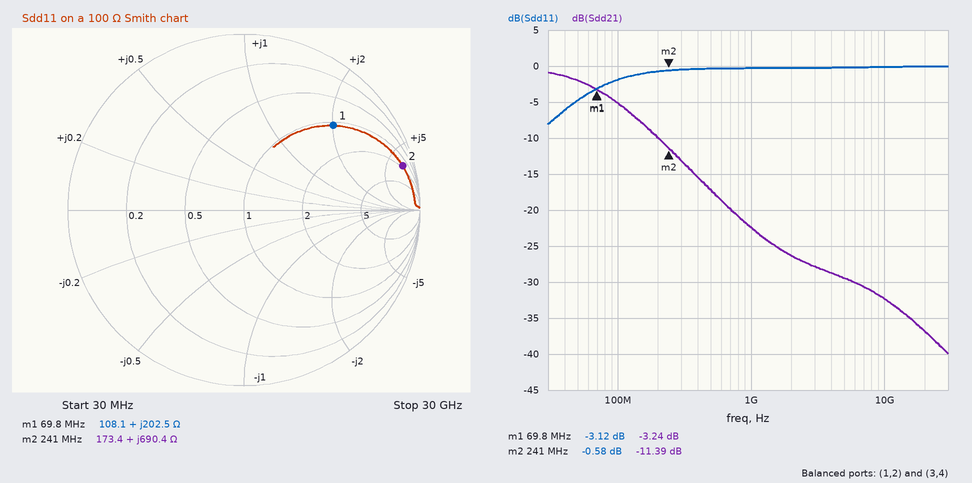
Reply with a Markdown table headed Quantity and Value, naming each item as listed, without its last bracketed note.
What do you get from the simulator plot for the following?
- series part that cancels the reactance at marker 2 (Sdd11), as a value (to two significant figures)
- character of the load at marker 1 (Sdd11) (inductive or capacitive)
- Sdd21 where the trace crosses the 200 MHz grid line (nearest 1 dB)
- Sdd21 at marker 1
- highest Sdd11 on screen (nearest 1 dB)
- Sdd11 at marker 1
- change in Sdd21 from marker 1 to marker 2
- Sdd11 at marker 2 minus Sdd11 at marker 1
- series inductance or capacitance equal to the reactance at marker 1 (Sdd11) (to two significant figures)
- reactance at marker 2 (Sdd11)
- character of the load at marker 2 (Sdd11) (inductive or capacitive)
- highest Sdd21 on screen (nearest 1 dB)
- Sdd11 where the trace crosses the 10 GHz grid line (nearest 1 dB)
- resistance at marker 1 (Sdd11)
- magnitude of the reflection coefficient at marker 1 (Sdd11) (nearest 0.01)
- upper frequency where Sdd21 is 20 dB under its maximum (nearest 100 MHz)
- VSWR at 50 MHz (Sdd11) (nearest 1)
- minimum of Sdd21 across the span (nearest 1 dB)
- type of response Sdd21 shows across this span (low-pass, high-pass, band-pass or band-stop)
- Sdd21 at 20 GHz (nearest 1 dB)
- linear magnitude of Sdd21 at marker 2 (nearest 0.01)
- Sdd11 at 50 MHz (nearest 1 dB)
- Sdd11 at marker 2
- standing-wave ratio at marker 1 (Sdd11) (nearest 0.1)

| Quantity | Value |
|---|---|
| series part that cancels the reactance at marker 2 (Sdd11), as a value | 960 fF |
| character of the load at marker 1 (Sdd11) | inductive |
| Sdd21 where the trace crosses the 200 MHz grid line | -10 dB |
| Sdd21 at marker 1 | -3.24 dB |
| highest Sdd11 on screen | 0 dB |
| Sdd11 at marker 1 | -3.12 dB |
| change in Sdd21 from marker 1 to marker 2 | -8.15 dB |
| Sdd11 at marker 2 minus Sdd11 at marker 1 | 2.54 dB |
| series inductance or capacitance equal to the reactance at marker 1 (Sdd11) | 460 nH |
| reactance at marker 2 | +690.4 Ω |
| character of the load at marker 2 (Sdd11) | inductive |
| highest Sdd21 on screen | -1 dB |
| Sdd11 where the trace crosses the 10 GHz grid line | 0 dB |
| resistance at marker 1 | 108.1 Ω |
| magnitude of the reflection coefficient at marker 1 (Sdd11) | 0.70 |
| upper frequency where Sdd21 is 20 dB under its maximum | 800 MHz |
| VSWR at 50 MHz (Sdd11) | 4 |
| minimum of Sdd21 across the span | -40 dB |
| type of response Sdd21 shows across this span | low-pass |
| Sdd21 at 20 GHz | -37 dB |
| linear magnitude of Sdd21 at marker 2 | 0.27 |
| Sdd11 at 50 MHz | -5 dB |
| Sdd11 at marker 2 | -0.58 dB |
| standing-wave ratio at marker 1 (Sdd11) | 5.6 |
